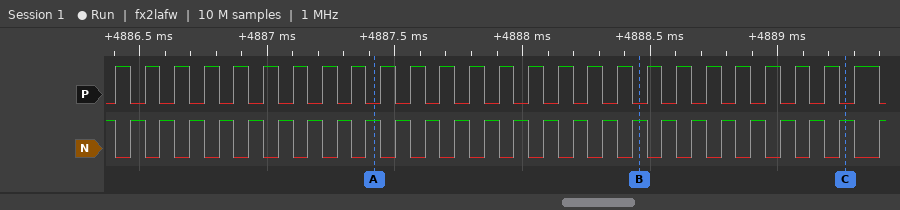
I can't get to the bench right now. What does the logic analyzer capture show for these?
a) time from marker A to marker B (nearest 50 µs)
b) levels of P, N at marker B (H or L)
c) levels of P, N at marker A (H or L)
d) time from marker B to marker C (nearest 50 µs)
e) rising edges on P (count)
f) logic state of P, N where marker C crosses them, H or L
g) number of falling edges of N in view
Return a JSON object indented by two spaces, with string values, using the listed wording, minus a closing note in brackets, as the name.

{
  "time from marker A to marker B": "1050 µs",
  "levels of P, N at marker B": "P=L, N=H",
  "levels of P, N at marker A": "P=L, N=H",
  "time from marker B to marker C": "800 µs",
  "rising edges on P": "26",
  "logic state of P, N where marker C crosses them, H or L": "P=L, N=H",
  "number of falling edges of N in view": "26"
}
